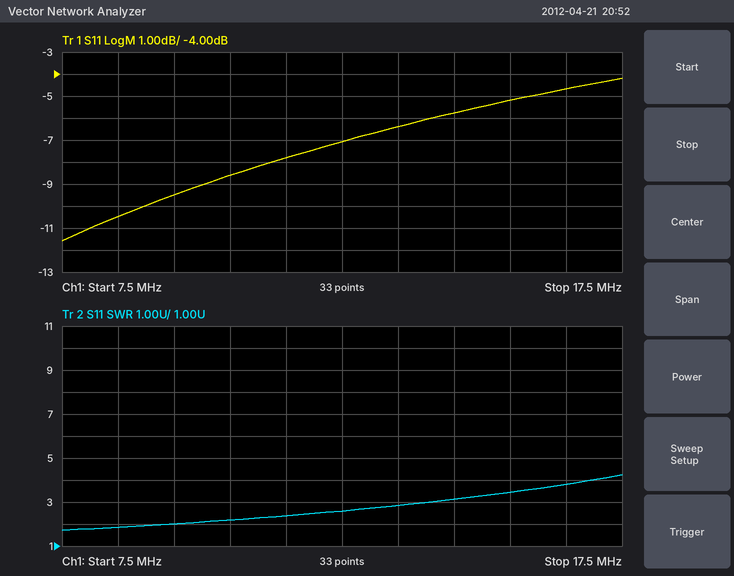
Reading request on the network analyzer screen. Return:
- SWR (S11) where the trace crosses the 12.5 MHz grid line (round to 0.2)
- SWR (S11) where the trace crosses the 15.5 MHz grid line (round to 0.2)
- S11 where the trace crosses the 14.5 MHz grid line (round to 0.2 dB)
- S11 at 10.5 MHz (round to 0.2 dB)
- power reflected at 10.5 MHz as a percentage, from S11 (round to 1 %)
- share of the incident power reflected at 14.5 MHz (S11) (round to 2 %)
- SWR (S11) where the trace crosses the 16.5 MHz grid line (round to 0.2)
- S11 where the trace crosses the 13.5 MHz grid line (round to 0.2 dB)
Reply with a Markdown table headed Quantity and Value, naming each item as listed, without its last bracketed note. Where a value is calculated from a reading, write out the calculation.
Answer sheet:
| Quantity | Value |
|---|---|
| SWR (S11) where the trace crosses the 12.5 MHz grid line | 2.6 |
| SWR (S11) where the trace crosses the 15.5 MHz grid line | 3.4 |
| S11 where the trace crosses the 14.5 MHz grid line | -5.8 dB |
| S11 at 10.5 MHz | -8.6 dB |
| power reflected at 10.5 MHz as a percentage, from S11 | 10^(-8.6/10) ≈ 14 % |
| share of the incident power reflected at 14.5 MHz (S11) | 10^(-5.8/10) ≈ 26 % |
| SWR (S11) where the trace crosses the 16.5 MHz grid line | 3.8 |
| S11 where the trace crosses the 13.5 MHz grid line | -6.4 dB |
